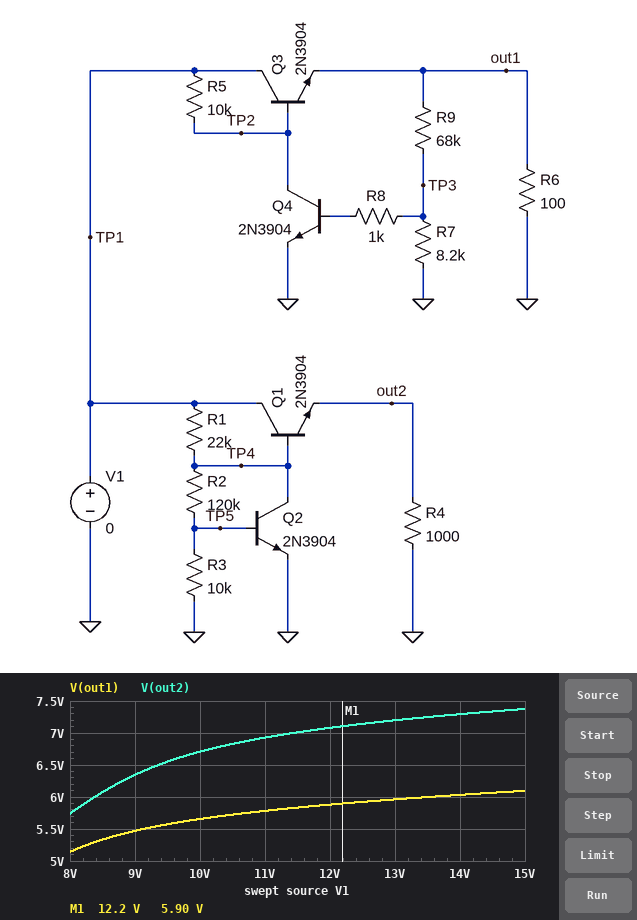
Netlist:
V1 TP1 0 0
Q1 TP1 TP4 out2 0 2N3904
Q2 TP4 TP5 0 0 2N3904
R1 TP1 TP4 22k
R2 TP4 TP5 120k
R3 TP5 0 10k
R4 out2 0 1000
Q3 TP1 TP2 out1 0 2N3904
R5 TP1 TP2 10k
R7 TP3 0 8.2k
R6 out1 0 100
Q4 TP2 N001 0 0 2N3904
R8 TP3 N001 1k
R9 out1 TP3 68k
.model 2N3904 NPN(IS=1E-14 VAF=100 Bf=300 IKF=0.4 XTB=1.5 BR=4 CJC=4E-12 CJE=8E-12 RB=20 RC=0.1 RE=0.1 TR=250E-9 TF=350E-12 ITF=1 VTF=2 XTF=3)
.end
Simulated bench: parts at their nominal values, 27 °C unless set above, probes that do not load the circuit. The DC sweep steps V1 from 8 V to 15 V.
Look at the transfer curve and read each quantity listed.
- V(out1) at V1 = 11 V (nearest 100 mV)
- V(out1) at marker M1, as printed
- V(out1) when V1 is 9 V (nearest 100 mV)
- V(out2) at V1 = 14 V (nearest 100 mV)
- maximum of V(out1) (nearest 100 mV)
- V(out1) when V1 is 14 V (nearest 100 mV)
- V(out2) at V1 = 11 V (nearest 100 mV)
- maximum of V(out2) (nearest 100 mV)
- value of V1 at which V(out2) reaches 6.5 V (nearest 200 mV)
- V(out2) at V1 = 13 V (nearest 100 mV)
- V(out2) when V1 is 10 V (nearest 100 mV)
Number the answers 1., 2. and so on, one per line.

1. 5.8 V
2. 5.90 V
3. 5.5 V
4. 7.3 V
5. 6.1 V
6. 6.0 V
7. 6.9 V
8. 7.4 V
9. 9.4 V
10. 7.2 V
11. 6.7 V
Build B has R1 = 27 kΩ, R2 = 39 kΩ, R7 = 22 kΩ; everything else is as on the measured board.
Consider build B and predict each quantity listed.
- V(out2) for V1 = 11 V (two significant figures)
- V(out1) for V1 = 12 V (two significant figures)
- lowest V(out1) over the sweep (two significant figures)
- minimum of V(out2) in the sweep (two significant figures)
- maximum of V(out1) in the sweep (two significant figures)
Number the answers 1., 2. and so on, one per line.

1. 2.4 V
2. 2.8 V
3. 2.7 V
4. 2.3 V
5. 2.9 V
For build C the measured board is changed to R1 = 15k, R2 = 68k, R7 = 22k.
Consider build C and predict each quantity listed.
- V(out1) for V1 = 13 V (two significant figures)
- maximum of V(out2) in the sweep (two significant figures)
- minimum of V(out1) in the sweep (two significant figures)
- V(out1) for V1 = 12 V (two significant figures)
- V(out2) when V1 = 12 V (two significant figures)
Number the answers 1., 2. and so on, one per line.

1. 2.9 V
2. 4.4 V
3. 2.7 V
4. 2.8 V
5. 4.3 V
